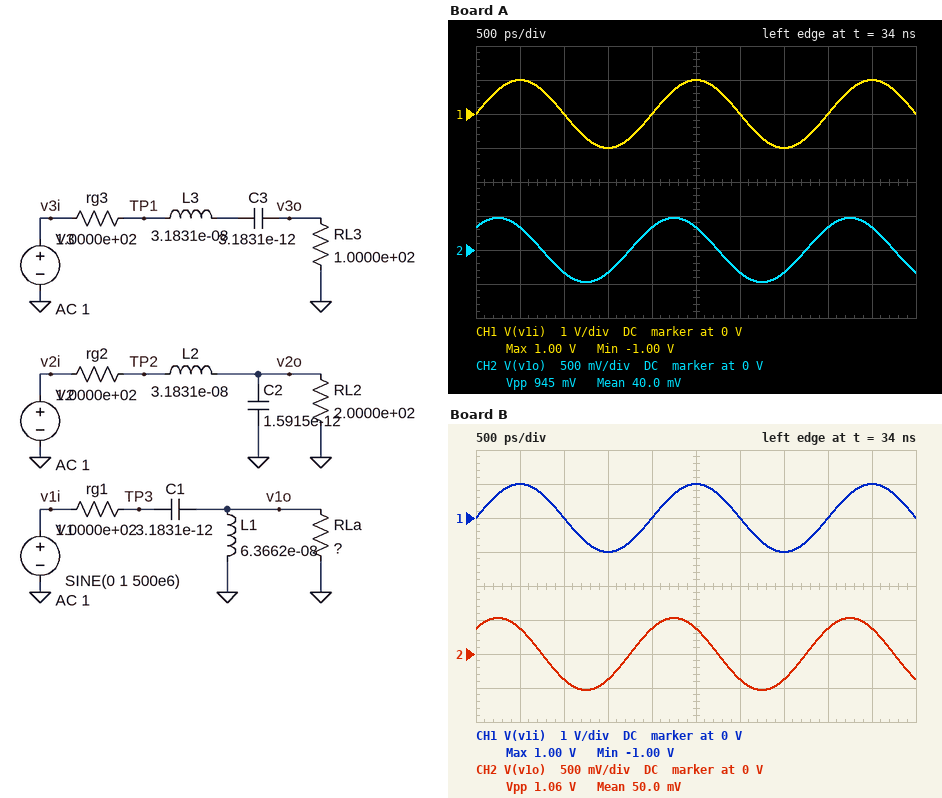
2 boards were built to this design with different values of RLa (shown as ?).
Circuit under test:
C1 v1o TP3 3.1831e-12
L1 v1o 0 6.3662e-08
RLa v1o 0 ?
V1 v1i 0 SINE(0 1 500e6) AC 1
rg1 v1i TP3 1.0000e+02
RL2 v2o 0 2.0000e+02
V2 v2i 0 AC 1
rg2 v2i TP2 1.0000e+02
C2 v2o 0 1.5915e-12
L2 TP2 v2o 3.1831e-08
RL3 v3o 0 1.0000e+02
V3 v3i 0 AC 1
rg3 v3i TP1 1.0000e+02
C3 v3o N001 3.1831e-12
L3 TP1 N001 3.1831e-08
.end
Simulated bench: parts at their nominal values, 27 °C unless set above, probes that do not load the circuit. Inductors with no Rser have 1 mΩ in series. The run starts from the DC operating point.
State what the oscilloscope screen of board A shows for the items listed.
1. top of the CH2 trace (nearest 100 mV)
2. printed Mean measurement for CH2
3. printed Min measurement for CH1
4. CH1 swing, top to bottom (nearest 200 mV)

500 mV
40.0 mV
-1.00 V
2.0 V
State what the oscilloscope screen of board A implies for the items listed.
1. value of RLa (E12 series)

100 Ω
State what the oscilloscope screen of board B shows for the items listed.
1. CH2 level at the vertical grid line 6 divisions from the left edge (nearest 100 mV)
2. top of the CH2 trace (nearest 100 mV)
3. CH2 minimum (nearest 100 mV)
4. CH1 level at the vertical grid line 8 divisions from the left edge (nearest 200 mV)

-400 mV
500 mV
-500 mV
0 V
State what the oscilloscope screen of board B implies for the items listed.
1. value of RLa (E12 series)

120 Ω
